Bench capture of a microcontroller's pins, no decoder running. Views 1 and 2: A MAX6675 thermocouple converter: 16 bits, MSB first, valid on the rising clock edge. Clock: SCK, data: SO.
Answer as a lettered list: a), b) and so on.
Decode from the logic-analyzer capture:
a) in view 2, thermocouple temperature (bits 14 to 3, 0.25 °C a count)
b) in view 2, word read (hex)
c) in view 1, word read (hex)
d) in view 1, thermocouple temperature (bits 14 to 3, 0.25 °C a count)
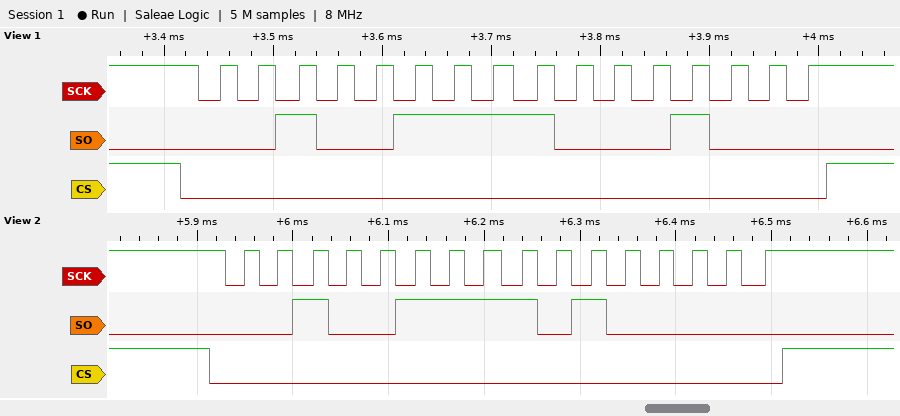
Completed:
a) 317.00 °C
b) 0x27A0
c) 0x2788
d) 316.25 °C
